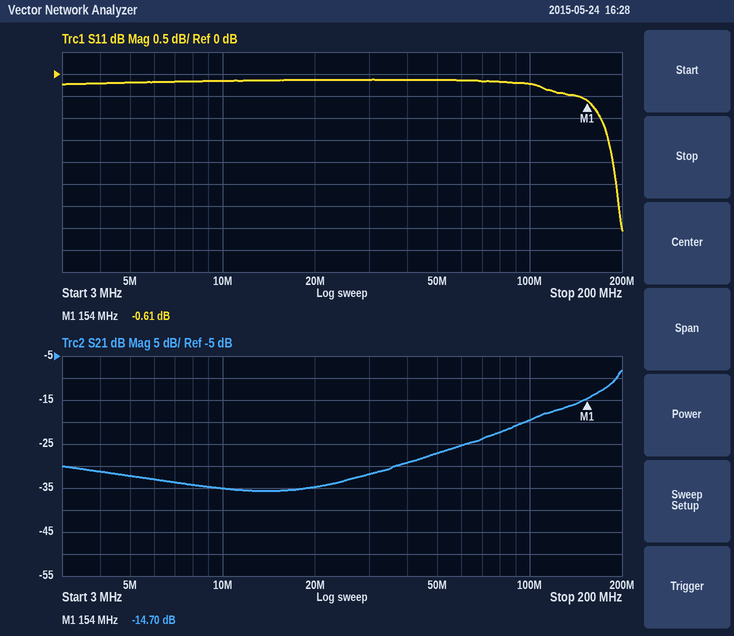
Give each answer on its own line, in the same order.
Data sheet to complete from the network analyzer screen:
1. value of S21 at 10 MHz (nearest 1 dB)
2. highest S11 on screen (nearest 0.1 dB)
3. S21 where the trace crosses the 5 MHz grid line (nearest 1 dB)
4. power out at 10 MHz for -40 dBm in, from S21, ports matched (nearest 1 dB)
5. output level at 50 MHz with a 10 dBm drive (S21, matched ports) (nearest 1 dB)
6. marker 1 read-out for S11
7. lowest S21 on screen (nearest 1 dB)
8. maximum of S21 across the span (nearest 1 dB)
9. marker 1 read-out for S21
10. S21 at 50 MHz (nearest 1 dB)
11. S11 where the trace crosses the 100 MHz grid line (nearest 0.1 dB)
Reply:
-35 dB
-0.1 dB
-32 dB
-75 dBm
-17 dBm
-0.61 dB
-36 dB
-8 dB
-14.70 dB
-27 dB
-0.2 dB
